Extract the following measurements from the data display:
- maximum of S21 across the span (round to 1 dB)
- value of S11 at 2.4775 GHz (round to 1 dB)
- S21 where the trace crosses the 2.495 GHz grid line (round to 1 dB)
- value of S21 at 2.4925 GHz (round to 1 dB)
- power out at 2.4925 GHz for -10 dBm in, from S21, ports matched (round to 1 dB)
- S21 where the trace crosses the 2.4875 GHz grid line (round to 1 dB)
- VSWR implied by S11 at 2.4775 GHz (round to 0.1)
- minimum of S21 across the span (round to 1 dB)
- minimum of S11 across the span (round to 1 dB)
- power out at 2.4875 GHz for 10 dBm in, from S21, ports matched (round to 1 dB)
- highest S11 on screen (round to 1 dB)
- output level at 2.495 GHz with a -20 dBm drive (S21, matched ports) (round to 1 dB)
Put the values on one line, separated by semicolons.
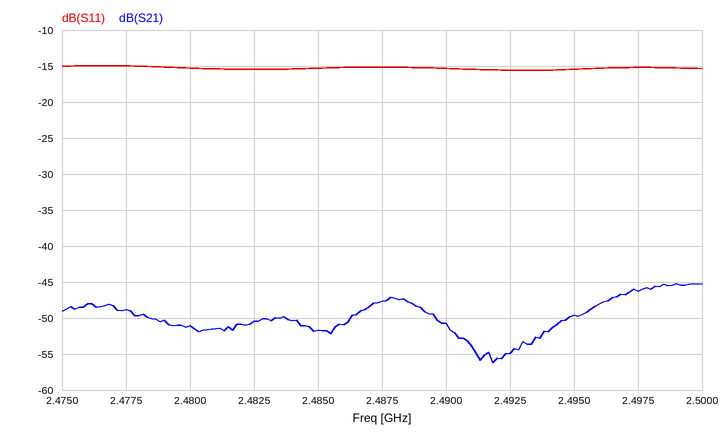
-45 dB; -15 dB; -50 dB; -55 dB; -65 dBm; -48 dB; 1.4; -56 dB; -16 dB; -38 dBm; -15 dB; -70 dBm
